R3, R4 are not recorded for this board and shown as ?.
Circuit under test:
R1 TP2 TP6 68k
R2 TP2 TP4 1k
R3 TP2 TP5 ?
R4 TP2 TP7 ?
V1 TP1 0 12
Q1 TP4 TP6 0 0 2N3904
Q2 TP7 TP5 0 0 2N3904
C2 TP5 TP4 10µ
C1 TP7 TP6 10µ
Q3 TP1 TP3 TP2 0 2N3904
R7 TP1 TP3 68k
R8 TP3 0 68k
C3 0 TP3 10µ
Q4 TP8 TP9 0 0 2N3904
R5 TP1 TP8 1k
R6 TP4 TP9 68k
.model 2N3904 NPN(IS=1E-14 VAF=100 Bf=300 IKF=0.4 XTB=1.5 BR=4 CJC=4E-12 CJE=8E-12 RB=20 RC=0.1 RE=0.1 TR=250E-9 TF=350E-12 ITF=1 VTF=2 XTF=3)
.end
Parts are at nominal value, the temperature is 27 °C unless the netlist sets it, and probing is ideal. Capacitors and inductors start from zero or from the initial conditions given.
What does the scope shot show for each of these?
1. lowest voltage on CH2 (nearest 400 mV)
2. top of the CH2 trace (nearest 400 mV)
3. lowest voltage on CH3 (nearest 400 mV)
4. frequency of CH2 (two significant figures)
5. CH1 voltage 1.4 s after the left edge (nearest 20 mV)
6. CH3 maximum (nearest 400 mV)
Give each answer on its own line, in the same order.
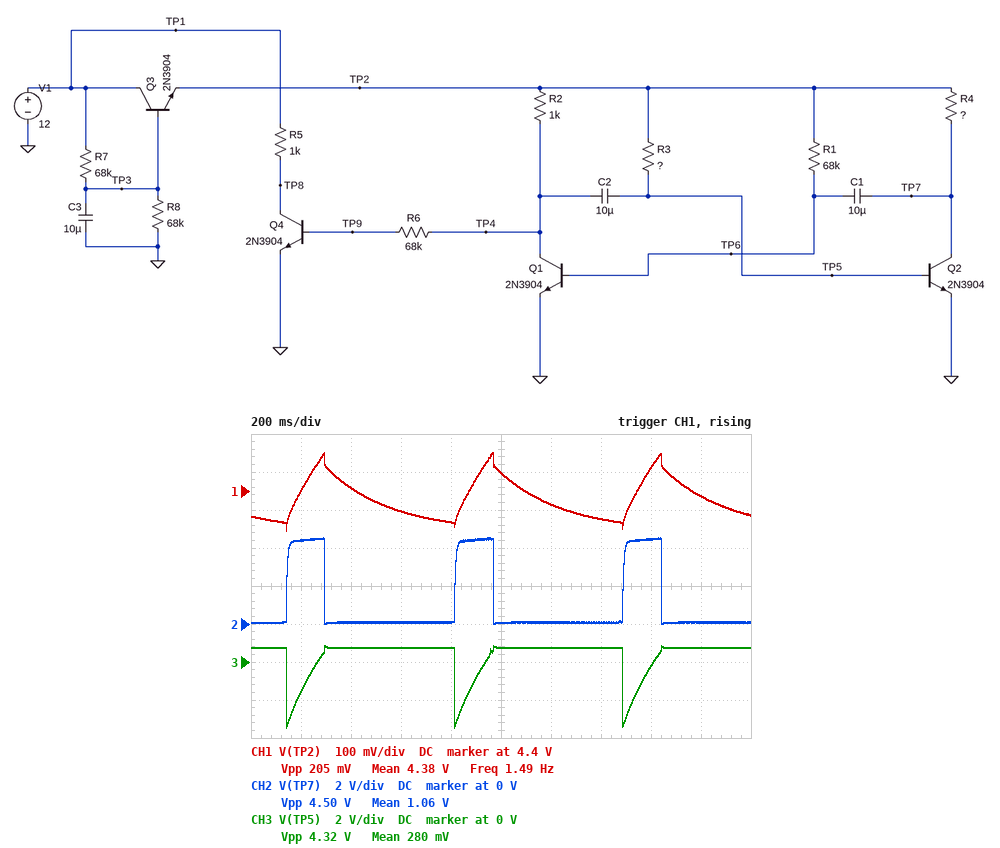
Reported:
0 V
4.4 V
-3.6 V
1.5 Hz
4.32 V
800 mV
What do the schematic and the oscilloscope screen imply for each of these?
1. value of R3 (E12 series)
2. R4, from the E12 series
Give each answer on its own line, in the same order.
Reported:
22 kΩ
470 Ω
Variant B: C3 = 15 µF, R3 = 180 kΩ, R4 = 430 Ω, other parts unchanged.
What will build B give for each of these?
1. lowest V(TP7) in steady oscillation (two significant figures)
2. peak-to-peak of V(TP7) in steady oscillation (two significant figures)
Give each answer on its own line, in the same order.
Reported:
20 mV
4.8 V
